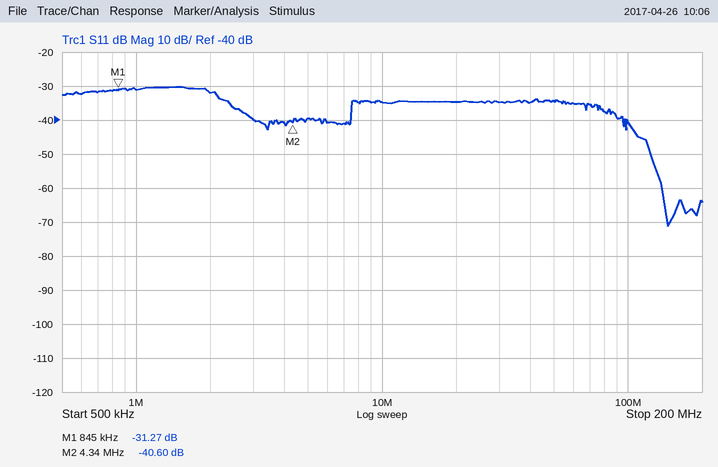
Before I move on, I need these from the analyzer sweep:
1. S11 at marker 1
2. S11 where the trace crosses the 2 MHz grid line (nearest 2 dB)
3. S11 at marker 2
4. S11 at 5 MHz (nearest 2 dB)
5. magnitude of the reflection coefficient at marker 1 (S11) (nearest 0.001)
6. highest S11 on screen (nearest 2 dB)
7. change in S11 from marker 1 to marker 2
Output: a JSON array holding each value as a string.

["-31.27 dB", "-32 dB", "-40.60 dB", "-40 dB", "0.027", "-30 dB", "-9.33 dB"]
